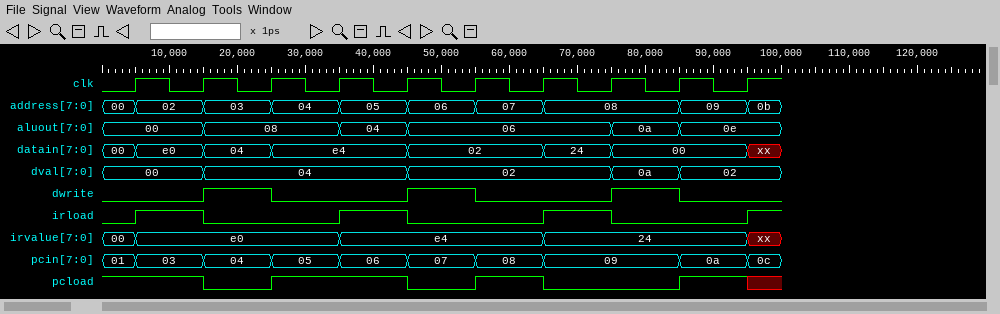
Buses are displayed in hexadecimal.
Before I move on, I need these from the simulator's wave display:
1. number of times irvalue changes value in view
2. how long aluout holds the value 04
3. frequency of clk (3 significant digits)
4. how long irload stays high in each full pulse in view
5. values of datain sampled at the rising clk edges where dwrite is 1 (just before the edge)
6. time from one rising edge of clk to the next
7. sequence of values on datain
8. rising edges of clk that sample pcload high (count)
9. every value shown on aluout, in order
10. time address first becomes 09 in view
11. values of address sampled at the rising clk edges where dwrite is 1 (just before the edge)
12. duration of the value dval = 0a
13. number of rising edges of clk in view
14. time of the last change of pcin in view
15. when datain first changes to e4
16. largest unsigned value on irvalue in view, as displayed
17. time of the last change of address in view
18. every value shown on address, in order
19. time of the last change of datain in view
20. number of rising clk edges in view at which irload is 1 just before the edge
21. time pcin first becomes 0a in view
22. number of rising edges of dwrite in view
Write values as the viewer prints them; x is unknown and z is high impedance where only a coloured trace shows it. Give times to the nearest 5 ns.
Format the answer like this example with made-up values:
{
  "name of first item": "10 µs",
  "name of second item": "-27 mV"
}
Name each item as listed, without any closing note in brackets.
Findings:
{
  "number of times irvalue changes value in view": "4",
  "how long aluout holds the value 04": "10 ns",
  "frequency of clk": "100 MHz",
  "how long irload stays high in each full pulse in view": "10 ns, 10 ns, 10 ns",
  "values of datain sampled at the rising clk edges where dwrite is 1": "04, 02, 00",
  "time from one rising edge of clk to the next": "10 ns",
  "sequence of values on datain": "00, e0, 04, e4, 02, 24, 00, xx",
  "rising edges of clk that sample pcload high": "6",
  "every value shown on aluout, in order": "00, 08, 04, 06, 0a, 0e",
  "time address first becomes 09 in view": "85 ns",
  "values of address sampled at the rising clk edges where dwrite is 1": "03, 06, 08",
  "duration of the value dval = 0a": "10 ns",
  "number of rising edges of clk in view": "10",
  "time of the last change of pcin in view": "95 ns",
  "when datain first changes to e4": "25 ns",
  "largest unsigned value on irvalue in view, as displayed": "e4",
  "time of the last change of address in view": "95 ns",
  "every value shown on address, in order": "00, 02, 03, 04, 05, 06, 07, 08, 09, 0b",
  "time of the last change of datain in view": "95 ns",
  "number of rising clk edges in view at which irload is 1 just before the edge": "3",
  "time pcin first becomes 0a in view": "85 ns",
  "number of rising edges of dwrite in view": "3"
}
